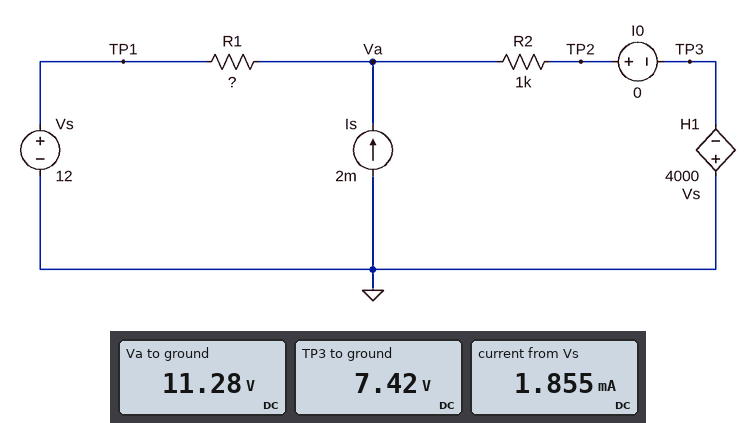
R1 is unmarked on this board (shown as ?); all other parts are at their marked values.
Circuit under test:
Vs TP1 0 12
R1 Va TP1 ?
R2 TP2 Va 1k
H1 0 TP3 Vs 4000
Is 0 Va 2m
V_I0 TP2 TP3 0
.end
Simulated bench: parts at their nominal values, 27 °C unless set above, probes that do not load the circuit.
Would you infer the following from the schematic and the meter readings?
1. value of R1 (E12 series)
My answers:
390 Ω
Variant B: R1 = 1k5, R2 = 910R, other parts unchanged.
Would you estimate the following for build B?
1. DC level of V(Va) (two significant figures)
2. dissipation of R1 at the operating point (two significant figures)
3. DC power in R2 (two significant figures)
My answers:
9.6 V
3.8 mW
12 mW
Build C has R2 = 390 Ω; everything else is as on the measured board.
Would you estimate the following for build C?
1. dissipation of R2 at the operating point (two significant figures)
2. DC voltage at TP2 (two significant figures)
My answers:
7.4 mW
9.4 V
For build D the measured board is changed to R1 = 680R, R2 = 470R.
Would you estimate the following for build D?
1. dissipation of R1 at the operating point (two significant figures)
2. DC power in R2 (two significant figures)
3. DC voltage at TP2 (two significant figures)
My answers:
3.1 mW
8.1 mW
8.6 V
